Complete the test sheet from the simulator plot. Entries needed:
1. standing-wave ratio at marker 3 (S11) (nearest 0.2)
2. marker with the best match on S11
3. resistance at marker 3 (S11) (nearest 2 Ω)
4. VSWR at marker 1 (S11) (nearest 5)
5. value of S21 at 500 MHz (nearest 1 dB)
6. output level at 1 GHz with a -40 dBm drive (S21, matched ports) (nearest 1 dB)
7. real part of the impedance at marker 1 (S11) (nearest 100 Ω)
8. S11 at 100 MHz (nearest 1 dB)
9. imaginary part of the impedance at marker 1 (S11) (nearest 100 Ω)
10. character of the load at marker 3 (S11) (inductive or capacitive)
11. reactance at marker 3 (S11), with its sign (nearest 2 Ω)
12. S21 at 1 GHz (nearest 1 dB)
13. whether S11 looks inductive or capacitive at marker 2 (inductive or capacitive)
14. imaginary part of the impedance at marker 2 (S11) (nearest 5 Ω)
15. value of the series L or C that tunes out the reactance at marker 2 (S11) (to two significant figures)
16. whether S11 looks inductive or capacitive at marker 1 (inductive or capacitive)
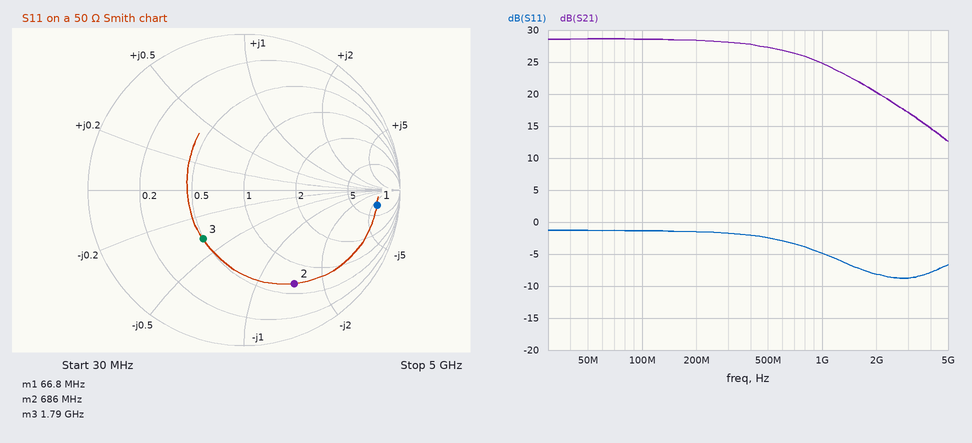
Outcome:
2.4
marker 3
24 Ω
15
27 dB
-15 dBm
400 Ω
-1 dB
-300 Ω
capacitive
-18 Ω
25 dB
capacitive
-75 Ω
17 nH
capacitive
